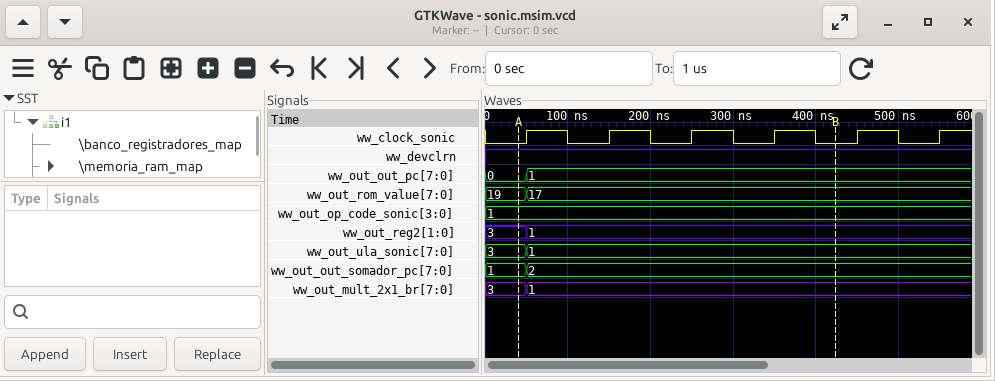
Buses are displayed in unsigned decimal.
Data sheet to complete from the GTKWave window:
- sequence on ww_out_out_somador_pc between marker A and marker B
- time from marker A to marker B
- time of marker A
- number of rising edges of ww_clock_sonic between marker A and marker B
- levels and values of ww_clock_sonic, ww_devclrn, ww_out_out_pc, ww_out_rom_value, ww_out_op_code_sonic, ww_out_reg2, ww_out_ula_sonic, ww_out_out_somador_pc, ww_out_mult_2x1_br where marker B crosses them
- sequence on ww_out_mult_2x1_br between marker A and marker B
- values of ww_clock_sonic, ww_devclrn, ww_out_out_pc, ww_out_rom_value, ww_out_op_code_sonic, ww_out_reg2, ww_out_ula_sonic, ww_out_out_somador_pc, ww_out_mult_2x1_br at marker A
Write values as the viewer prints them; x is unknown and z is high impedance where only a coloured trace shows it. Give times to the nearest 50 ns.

1, 2
400 ns
50 ns
4
ww_clock_sonic=0, ww_devclrn=1, ww_out_out_pc=1, ww_out_rom_value=17, ww_out_op_code_sonic=1, ww_out_reg2=1, ww_out_ula_sonic=1, ww_out_out_somador_pc=2, ww_out_mult_2x1_br=1
3, 1
ww_clock_sonic=0, ww_devclrn=1, ww_out_out_pc=0, ww_out_rom_value=19, ww_out_op_code_sonic=1, ww_out_reg2=3, ww_out_ula_sonic=3, ww_out_out_somador_pc=1, ww_out_mult_2x1_br=3
